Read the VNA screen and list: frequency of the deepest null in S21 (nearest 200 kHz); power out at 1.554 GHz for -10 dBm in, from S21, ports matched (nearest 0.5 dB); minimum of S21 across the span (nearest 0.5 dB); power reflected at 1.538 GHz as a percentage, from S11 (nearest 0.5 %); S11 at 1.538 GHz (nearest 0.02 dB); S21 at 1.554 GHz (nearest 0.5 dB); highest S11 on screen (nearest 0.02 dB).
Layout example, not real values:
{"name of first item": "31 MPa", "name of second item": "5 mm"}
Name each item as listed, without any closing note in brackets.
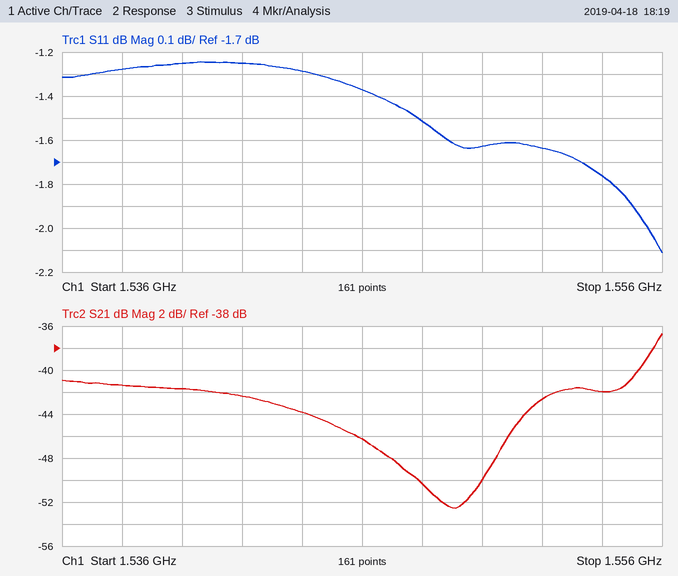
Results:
{"frequency of the deepest null in S21": "1.5492 GHz", "power out at 1.554 GHz for -10 dBm in, from S21, ports matched": "-52.0 dBm", "minimum of S21 across the span": "-52.5 dB", "power reflected at 1.538 GHz as a percentage, from S11": "74.5 %", "S11 at 1.538 GHz": "-1.28 dB", "S21 at 1.554 GHz": "-42.0 dB", "highest S11 on screen": "-1.24 dB"}
